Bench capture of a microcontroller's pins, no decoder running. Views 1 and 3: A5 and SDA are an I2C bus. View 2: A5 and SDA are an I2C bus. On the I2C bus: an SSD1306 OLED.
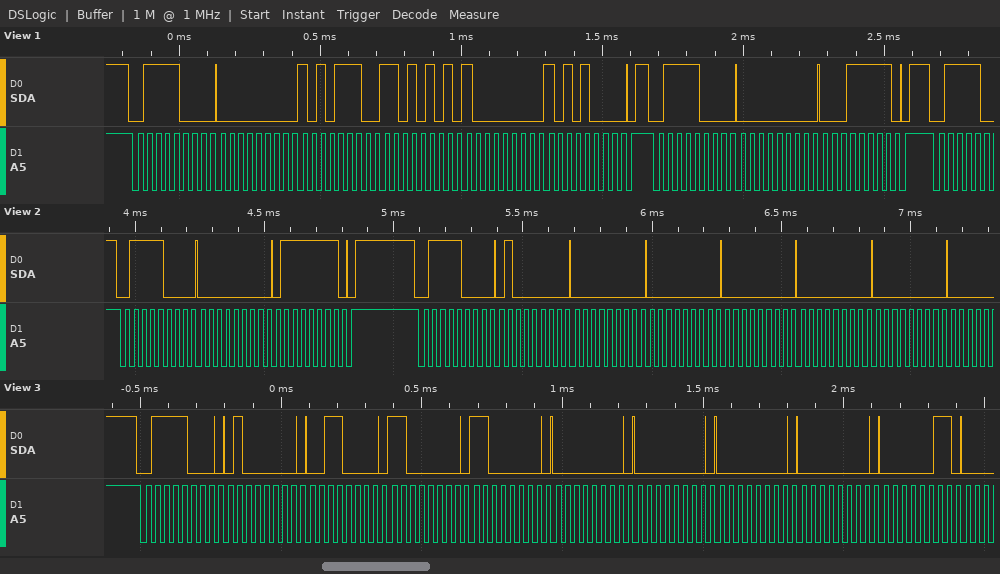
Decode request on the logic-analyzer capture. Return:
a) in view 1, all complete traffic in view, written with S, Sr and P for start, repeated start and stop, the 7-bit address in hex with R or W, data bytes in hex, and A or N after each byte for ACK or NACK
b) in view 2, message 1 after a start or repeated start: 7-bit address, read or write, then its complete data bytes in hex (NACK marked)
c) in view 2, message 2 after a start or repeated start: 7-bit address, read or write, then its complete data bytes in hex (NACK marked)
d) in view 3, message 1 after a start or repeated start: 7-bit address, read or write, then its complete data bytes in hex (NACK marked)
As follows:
S 3CW A 00 A AE A D5 A 80 A A8 A P S 3CW A 00 A 1F A P
0x3C write: 00 7F
0x3C write: 40 00 00 00 00 00
0x3C write: 40 30 C0 C0 00 00 00 00 03
